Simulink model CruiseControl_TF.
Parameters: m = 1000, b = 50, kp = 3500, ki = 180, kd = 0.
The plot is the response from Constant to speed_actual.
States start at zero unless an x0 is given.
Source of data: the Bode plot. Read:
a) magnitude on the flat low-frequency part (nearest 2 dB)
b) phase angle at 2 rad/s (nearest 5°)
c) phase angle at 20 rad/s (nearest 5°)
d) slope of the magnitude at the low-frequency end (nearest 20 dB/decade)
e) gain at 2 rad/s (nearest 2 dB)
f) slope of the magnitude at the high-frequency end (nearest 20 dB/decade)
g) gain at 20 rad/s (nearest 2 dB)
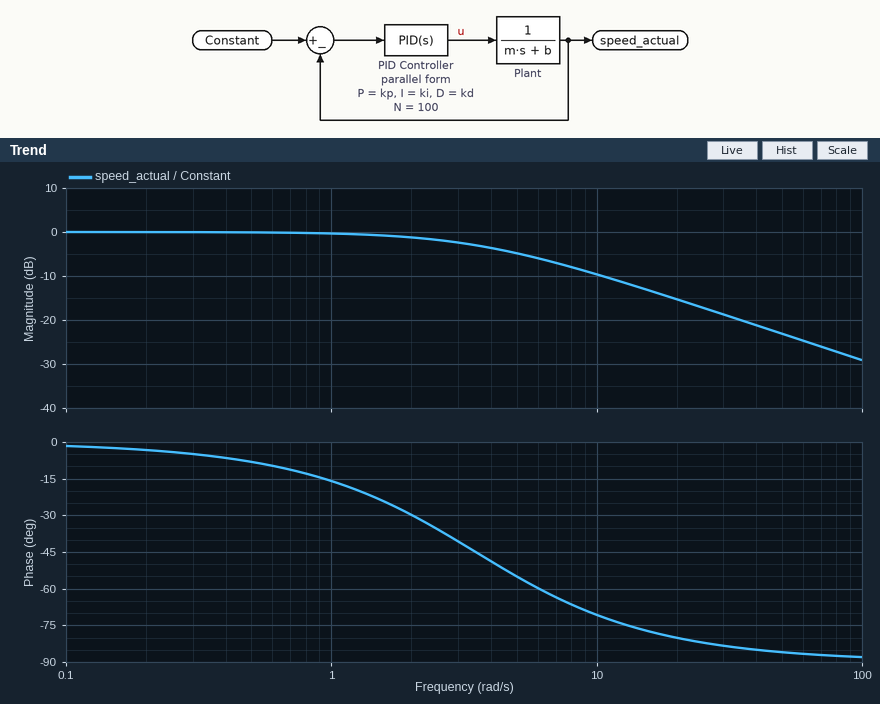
0 dB
-30°
-80°
0 dB/decade
-2 dB
-20 dB/decade
-16 dB
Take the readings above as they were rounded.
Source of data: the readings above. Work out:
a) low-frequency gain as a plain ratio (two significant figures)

1.0
